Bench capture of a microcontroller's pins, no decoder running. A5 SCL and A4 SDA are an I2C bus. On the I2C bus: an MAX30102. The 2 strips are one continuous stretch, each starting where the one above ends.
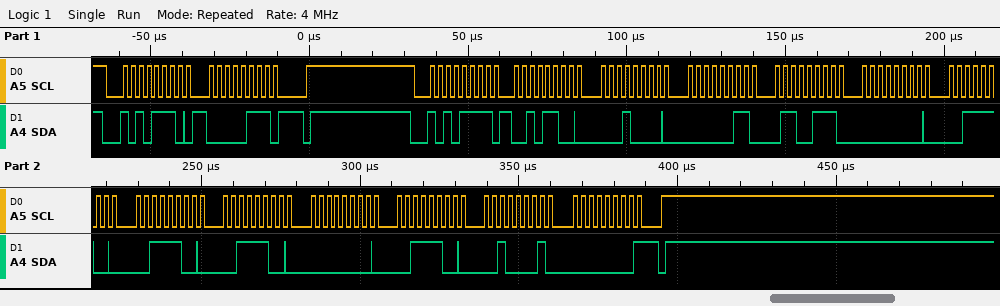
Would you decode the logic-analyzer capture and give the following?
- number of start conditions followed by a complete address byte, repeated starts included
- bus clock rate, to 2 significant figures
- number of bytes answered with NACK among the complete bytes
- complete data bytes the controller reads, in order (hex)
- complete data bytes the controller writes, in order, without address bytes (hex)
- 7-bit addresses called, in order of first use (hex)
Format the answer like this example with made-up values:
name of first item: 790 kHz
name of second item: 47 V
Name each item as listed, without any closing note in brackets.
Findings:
number of start conditions followed by a complete address byte, repeated starts included: 2
bus clock rate, to 2 significant figures: 400 kHz
number of bytes answered with NACK among the complete bytes: 1
complete data bytes the controller reads, in order: 2C 10 03 67 00 3C 3C 3C 00 3C 21 00
complete data bytes the controller writes, in order, without address bytes: 07
7-bit addresses called, in order of first use: 0x57
